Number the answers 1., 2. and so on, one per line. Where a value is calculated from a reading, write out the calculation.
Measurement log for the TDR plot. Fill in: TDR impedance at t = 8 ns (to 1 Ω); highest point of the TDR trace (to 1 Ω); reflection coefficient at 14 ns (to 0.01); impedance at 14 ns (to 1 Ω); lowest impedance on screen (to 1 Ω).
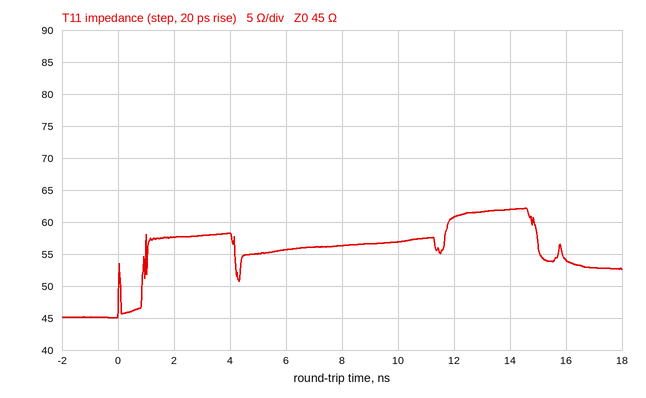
1. 56 Ω
2. 62 Ω
3. (62 − 45)/(62 + 45) ≈ +0.16
4. 62 Ω
5. 45 Ω
